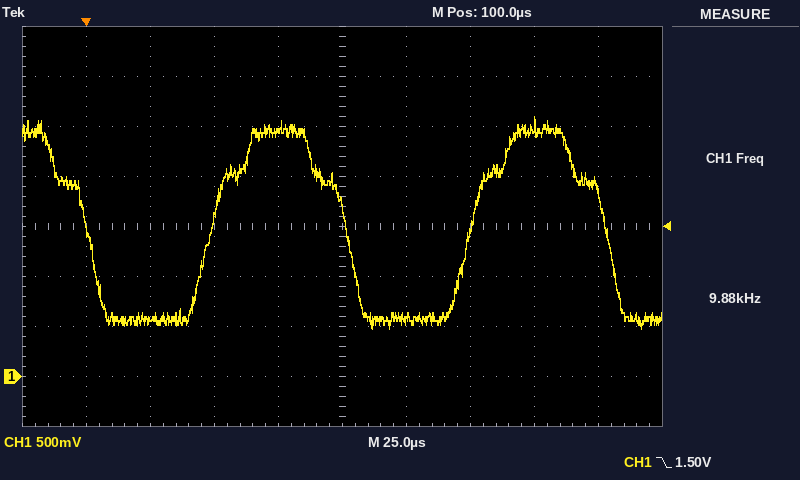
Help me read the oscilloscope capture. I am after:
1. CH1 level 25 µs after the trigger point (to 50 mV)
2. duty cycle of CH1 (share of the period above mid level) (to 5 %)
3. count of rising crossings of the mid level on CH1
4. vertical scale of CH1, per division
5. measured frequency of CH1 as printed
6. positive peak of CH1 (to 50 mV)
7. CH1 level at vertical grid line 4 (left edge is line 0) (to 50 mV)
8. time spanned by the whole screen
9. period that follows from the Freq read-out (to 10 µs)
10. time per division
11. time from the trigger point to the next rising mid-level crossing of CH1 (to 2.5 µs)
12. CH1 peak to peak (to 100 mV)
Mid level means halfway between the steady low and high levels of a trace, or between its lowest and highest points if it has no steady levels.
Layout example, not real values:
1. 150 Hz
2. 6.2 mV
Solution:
1. 550 mV
2. 50 %
3. 2
4. 500 mV
5. 9.88 kHz
6. 2.60 V
7. 2.45 V
8. 250 µs
9. 100 µs
10. 25 µs
11. 50.0 µs
12. 2.10 V
